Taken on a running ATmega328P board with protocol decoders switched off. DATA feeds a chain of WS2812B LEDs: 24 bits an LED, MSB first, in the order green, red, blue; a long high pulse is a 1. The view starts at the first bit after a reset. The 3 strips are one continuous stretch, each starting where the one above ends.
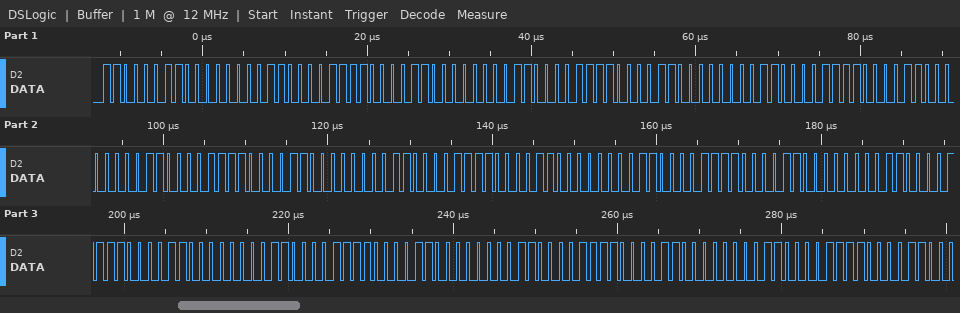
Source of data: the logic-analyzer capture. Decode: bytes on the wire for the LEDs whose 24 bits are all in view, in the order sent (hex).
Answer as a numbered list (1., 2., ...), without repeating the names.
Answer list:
1. C3 00 C3 C3 00 C3 C3 00 C3 C3 00 C3 C3 00 C3 C3 00 C3 C3 00 C3 C3 00 C3 C3 00 C3 C3 00 C3
